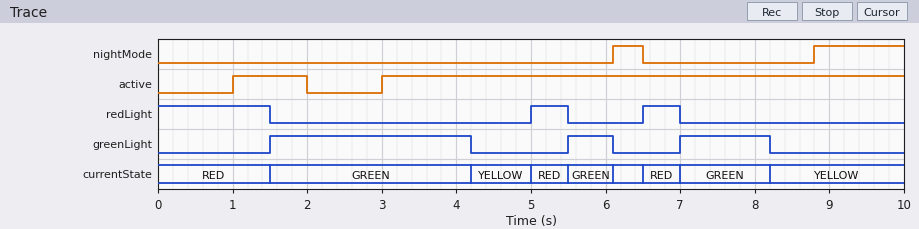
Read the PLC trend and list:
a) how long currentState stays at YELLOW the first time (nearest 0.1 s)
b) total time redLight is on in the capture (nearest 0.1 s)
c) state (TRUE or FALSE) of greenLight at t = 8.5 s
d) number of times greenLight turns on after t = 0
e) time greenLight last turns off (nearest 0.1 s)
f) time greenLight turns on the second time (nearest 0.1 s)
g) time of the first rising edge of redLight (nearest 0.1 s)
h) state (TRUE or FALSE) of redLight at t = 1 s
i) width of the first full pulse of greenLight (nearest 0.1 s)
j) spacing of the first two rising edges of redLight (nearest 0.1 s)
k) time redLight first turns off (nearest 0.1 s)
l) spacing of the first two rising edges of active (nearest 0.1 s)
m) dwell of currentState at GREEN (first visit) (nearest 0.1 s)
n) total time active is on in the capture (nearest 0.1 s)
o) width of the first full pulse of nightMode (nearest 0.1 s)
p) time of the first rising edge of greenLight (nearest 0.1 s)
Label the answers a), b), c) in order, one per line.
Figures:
a) 0.8 s
b) 2.5 s
c) FALSE
d) 3
e) 8.2 s
f) 5.5 s
g) 5.0 s
h) TRUE
i) 2.7 s
j) 1.5 s
k) 1.5 s
l) 2.0 s
m) 2.7 s
n) 8.0 s
o) 0.4 s
p) 1.5 s
